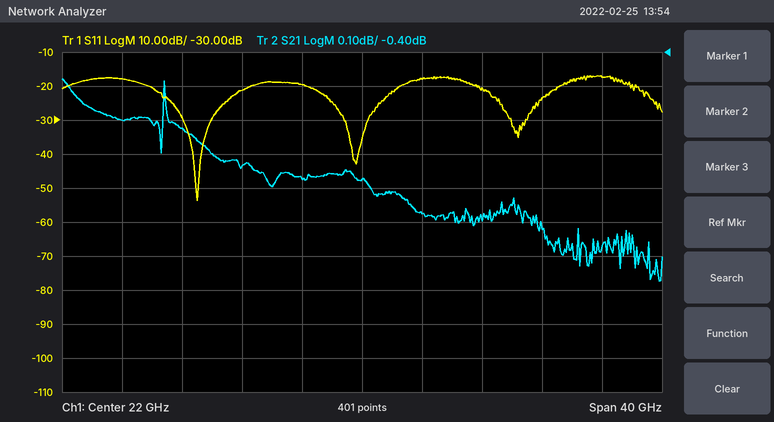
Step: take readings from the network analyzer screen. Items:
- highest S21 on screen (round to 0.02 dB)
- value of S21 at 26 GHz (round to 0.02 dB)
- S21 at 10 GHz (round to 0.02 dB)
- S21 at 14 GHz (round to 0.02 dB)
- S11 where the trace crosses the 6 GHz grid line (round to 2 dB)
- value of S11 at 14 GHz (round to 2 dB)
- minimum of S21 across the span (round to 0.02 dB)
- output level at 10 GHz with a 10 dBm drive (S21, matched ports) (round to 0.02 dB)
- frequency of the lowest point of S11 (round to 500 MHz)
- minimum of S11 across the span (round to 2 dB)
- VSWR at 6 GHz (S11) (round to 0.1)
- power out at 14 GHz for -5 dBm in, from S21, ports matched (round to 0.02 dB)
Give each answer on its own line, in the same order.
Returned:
-0.48 dB
-0.88 dB
-0.62 dB
-0.74 dB
-18 dB
-22 dB
-1.08 dB
9.38 dBm
11.0 GHz
-54 dB
1.3
-5.74 dBm
